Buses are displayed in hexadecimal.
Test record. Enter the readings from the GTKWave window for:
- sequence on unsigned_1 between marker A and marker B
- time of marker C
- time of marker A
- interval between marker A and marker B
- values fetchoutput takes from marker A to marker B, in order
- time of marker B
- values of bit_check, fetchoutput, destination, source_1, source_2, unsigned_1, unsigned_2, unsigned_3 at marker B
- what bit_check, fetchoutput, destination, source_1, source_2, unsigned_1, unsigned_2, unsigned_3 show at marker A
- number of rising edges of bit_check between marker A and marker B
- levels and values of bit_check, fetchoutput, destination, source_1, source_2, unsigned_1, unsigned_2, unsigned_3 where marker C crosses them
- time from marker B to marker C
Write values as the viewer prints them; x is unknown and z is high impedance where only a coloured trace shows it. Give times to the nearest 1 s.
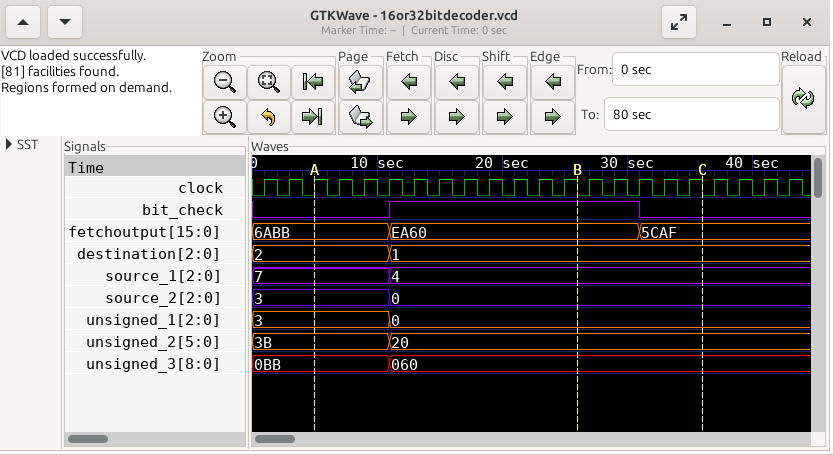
3, 0
36 s
5 s
21 s
6ABB, EA60
26 s
bit_check=1, fetchoutput=EA60, destination=1, source_1=4, source_2=0, unsigned_1=0, unsigned_2=20, unsigned_3=060
bit_check=0, fetchoutput=6ABB, destination=2, source_1=7, source_2=3, unsigned_1=3, unsigned_2=3B, unsigned_3=0BB
1
bit_check=0, fetchoutput=5CAF, destination=1, source_1=4, source_2=0, unsigned_1=0, unsigned_2=20, unsigned_3=060
10 s
